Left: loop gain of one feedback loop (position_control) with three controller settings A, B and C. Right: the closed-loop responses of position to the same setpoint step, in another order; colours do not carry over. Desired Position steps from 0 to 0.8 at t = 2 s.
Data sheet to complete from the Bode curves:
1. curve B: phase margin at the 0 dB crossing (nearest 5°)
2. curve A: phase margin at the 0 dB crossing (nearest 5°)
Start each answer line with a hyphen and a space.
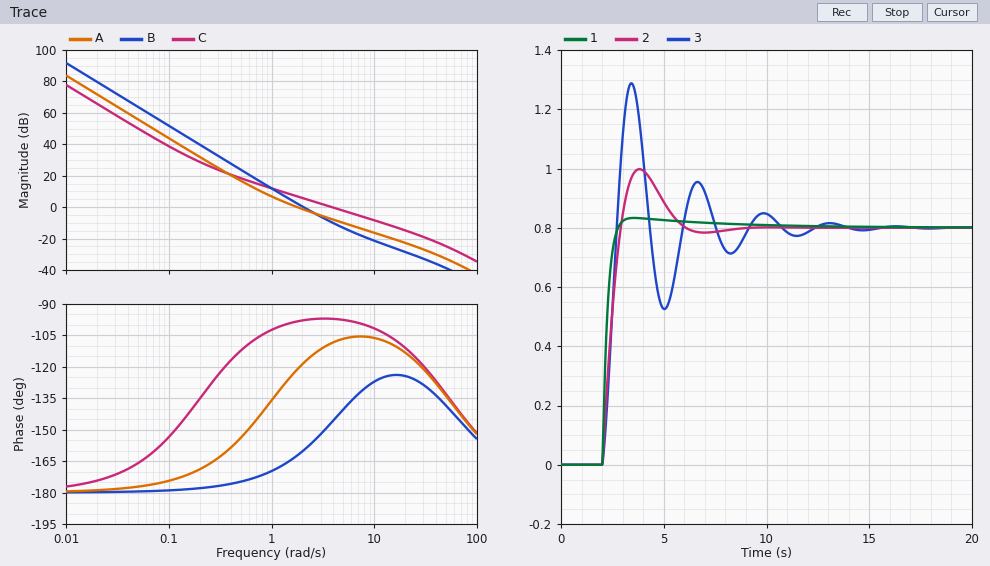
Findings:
- 20°
- 60°
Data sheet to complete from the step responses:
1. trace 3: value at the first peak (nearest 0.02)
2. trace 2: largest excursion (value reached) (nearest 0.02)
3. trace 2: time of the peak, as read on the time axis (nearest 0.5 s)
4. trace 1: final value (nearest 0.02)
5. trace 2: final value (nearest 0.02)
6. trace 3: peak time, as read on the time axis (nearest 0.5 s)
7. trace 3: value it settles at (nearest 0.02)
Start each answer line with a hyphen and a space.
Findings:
- 1.28
- 1.00
- 4.0 s
- 0.80
- 0.80
- 3.5 s
- 0.80
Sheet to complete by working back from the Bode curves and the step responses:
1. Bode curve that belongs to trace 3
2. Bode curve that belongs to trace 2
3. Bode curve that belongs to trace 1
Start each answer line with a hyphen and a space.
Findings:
- B
- A
- C
